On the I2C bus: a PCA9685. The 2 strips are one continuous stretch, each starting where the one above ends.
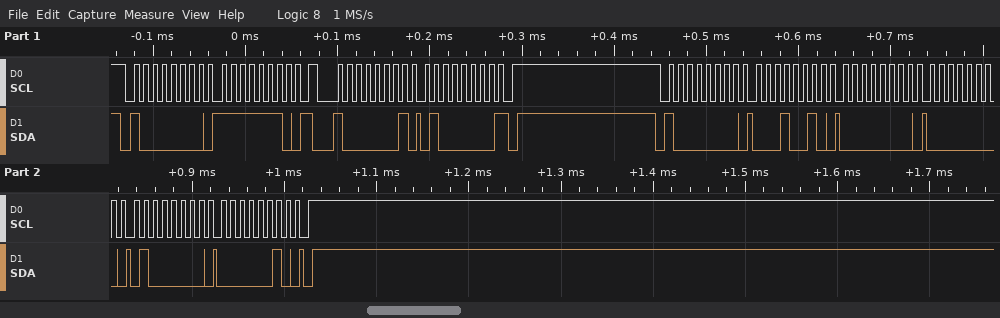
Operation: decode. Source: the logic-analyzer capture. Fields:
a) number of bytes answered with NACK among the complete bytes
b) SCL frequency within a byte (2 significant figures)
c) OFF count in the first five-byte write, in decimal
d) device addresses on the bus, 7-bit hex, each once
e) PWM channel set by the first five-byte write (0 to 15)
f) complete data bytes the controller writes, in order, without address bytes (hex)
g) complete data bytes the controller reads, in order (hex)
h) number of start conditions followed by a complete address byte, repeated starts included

1
100 kHz
576
0x40
3
FE 12 00 00 40 02
40
3
